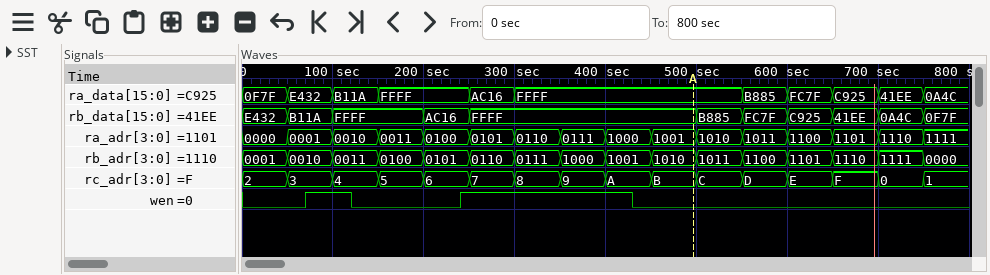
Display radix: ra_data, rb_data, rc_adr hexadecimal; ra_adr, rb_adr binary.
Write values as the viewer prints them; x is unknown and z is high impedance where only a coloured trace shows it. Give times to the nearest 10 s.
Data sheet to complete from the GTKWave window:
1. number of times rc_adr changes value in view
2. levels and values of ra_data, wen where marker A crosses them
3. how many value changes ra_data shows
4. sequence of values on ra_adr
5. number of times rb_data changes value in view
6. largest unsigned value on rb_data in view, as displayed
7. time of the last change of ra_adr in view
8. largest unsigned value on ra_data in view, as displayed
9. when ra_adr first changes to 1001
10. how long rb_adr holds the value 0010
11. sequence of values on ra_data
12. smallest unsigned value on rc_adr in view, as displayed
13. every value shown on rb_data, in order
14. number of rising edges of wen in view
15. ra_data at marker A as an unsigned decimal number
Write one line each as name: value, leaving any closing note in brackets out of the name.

number of times rc_adr changes value in view: 15
levels and values of ra_data, wen where marker A crosses them: ra_data=FFFF, wen=0
how many value changes ra_data shows: 10
sequence of values on ra_adr: 0000, 0001, 0010, 0011, 0100, 0101, 0110, 0111, 1000, 1001, 1010, 1011, 1100, 1101, 1110, 1111
number of times rb_data changes value in view: 10
largest unsigned value on rb_data in view, as displayed: FFFF
time of the last change of ra_adr in view: 750 s
largest unsigned value on ra_data in view, as displayed: FFFF
when ra_adr first changes to 1001: 450 s
how long rb_adr holds the value 0010: 50 s
sequence of values on ra_data: 0F7F, E432, B11A, FFFF, AC16, FFFF, B885, FC7F, C925, 41EE, 0A4C
smallest unsigned value on rc_adr in view, as displayed: 0
every value shown on rb_data, in order: E432, B11A, FFFF, AC16, FFFF, B885, FC7F, C925, 41EE, 0A4C, 0F7F
number of rising edges of wen in view: 2
ra_data at marker A as an unsigned decimal number: 65535
